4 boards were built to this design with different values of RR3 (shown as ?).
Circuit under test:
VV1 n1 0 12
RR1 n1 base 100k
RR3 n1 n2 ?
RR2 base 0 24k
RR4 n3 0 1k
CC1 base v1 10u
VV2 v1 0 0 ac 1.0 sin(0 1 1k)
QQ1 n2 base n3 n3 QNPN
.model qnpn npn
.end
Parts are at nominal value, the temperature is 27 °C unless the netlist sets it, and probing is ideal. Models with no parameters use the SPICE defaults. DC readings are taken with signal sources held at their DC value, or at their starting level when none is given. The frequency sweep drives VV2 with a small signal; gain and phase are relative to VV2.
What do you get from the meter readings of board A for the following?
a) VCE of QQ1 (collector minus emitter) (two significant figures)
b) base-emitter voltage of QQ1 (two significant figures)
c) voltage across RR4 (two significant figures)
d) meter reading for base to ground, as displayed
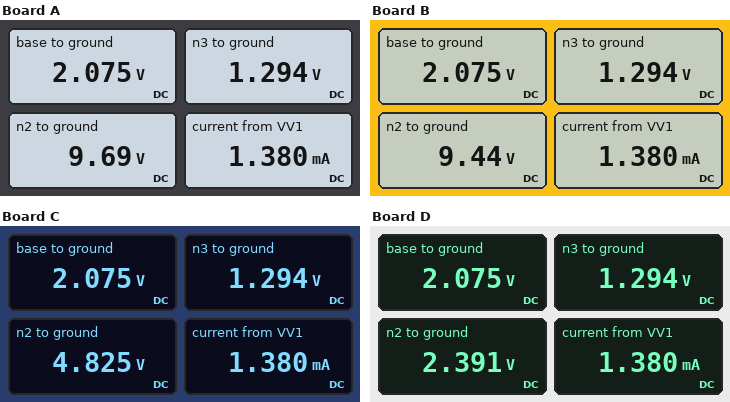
8.4 V
780 mV
1.3 V
2.075 V
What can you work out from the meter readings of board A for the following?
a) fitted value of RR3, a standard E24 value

1.8 kΩ
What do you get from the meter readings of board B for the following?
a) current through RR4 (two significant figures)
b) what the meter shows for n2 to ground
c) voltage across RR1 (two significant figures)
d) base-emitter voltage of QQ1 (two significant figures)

1.3 mA
9.44 V
9.9 V
780 mV
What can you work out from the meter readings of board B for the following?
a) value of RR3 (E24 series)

2 kΩ
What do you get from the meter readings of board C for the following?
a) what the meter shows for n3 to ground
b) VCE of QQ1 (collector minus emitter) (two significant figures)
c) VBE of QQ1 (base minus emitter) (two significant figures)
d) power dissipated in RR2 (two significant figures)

1.294 V
3.5 V
780 mV
180 µW
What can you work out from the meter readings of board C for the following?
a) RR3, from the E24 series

5.6 kΩ
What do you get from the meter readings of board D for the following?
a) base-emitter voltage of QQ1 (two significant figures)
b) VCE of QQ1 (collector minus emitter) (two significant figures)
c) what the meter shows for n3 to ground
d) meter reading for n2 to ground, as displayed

780 mV
1.1 V
1.294 V
2.391 V
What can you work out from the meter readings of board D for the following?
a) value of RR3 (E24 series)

7.5 kΩ
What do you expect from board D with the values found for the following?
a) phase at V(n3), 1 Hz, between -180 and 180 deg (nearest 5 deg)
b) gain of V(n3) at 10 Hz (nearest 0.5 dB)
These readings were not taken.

45 deg
0 dB
